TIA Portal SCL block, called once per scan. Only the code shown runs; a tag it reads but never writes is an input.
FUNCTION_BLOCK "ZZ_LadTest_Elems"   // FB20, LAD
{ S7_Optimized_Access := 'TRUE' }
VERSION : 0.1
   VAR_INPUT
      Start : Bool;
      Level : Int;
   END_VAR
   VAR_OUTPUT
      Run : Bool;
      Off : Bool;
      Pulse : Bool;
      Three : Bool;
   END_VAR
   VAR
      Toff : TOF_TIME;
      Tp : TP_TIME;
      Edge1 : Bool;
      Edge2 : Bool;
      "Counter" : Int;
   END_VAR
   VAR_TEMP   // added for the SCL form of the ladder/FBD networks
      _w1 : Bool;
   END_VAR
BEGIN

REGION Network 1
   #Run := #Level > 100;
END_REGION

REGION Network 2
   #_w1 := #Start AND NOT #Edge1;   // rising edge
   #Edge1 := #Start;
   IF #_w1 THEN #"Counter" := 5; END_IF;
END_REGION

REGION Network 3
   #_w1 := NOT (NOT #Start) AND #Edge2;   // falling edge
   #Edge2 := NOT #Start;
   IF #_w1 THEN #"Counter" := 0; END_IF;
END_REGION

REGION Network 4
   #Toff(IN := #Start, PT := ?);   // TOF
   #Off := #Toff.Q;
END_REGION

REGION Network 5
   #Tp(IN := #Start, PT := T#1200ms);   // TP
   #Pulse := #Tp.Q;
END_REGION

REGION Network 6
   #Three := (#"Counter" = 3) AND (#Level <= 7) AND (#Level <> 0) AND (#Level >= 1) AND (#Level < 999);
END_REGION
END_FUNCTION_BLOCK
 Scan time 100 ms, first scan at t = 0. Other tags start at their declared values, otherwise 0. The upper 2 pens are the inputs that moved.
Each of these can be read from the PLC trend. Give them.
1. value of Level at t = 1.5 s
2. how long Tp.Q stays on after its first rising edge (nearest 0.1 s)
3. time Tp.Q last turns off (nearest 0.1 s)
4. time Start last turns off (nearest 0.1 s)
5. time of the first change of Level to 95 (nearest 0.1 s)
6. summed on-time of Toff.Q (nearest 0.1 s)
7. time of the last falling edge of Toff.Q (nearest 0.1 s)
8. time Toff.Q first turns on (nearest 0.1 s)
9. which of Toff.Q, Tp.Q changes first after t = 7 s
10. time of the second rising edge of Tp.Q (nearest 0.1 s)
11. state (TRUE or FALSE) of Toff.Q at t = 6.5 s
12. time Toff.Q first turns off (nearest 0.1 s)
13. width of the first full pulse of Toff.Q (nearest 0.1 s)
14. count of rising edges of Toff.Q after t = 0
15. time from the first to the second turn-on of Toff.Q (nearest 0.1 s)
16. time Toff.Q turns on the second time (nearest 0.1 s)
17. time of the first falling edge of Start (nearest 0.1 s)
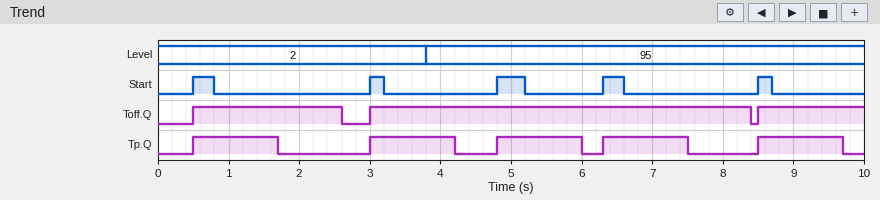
2
1.2 s
9.7 s
8.7 s
3.8 s
9.0 s
8.4 s
0.5 s
Tp.Q
3.0 s
TRUE
2.6 s
2.1 s
3
2.5 s
3.0 s
0.8 s
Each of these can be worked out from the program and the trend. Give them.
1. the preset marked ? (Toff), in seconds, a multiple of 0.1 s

1.8 s
